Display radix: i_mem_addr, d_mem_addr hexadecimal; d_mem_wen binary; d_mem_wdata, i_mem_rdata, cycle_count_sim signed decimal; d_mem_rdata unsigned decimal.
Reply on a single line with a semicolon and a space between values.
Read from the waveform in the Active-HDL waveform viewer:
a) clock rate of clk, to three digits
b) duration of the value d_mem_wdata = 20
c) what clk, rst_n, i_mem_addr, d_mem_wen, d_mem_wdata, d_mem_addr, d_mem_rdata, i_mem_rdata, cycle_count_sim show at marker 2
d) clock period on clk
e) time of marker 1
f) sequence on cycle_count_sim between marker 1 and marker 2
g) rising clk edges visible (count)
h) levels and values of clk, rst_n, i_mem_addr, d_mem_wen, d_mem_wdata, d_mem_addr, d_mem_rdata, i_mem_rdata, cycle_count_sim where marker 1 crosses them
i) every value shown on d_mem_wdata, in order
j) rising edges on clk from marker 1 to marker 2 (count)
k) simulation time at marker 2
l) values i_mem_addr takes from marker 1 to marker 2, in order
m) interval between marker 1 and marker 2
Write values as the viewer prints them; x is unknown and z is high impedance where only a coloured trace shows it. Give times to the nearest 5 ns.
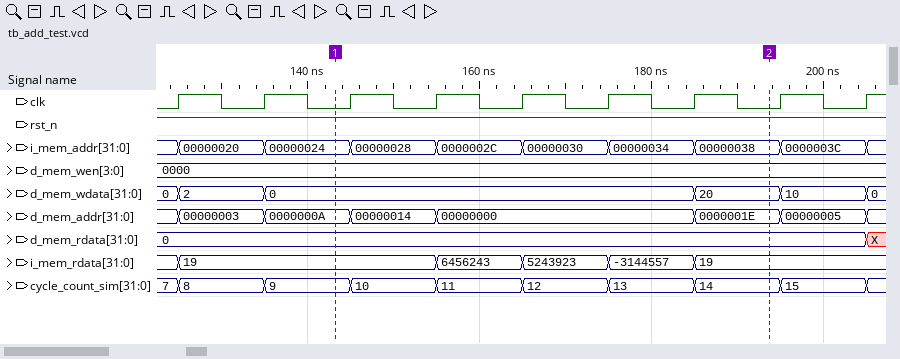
100 MHz; 10 ns; clk=0, rst_n=1, i_mem_addr=00000038, d_mem_wen=0000, d_mem_wdata=20, d_mem_addr=0000001E, d_mem_rdata=0, i_mem_rdata=19, cycle_count_sim=14; 10 ns; 145 ns; 9, 10, 11, 12, 13, 14; 9; clk=0, rst_n=1, i_mem_addr=00000024, d_mem_wen=0000, d_mem_wdata=0, d_mem_addr=0000000A, d_mem_rdata=0, i_mem_rdata=19, cycle_count_sim=9; 0, 2, 0, 20, 10, 0; 5; 195 ns; 00000024, 00000028, 0000002C, 00000030, 00000034, 00000038; 50 ns
